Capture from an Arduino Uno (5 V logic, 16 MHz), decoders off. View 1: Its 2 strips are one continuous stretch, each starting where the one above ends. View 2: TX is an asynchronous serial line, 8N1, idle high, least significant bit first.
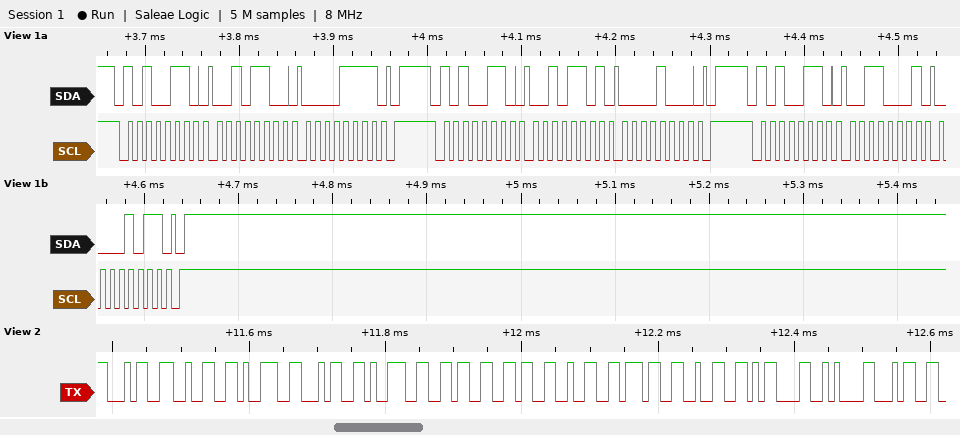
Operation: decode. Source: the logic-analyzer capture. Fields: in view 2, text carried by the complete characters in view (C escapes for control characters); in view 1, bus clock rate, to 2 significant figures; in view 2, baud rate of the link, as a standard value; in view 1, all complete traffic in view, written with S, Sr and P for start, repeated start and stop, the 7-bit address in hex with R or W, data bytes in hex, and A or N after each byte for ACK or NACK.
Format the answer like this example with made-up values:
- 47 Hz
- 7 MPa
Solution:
- "4294966272\r\n4"
- 100 kHz
- 115200 baud
- S 53W A 2C A 0F A P S 53W A 2D A 08 A P S 53W A 31 A 0B A P
